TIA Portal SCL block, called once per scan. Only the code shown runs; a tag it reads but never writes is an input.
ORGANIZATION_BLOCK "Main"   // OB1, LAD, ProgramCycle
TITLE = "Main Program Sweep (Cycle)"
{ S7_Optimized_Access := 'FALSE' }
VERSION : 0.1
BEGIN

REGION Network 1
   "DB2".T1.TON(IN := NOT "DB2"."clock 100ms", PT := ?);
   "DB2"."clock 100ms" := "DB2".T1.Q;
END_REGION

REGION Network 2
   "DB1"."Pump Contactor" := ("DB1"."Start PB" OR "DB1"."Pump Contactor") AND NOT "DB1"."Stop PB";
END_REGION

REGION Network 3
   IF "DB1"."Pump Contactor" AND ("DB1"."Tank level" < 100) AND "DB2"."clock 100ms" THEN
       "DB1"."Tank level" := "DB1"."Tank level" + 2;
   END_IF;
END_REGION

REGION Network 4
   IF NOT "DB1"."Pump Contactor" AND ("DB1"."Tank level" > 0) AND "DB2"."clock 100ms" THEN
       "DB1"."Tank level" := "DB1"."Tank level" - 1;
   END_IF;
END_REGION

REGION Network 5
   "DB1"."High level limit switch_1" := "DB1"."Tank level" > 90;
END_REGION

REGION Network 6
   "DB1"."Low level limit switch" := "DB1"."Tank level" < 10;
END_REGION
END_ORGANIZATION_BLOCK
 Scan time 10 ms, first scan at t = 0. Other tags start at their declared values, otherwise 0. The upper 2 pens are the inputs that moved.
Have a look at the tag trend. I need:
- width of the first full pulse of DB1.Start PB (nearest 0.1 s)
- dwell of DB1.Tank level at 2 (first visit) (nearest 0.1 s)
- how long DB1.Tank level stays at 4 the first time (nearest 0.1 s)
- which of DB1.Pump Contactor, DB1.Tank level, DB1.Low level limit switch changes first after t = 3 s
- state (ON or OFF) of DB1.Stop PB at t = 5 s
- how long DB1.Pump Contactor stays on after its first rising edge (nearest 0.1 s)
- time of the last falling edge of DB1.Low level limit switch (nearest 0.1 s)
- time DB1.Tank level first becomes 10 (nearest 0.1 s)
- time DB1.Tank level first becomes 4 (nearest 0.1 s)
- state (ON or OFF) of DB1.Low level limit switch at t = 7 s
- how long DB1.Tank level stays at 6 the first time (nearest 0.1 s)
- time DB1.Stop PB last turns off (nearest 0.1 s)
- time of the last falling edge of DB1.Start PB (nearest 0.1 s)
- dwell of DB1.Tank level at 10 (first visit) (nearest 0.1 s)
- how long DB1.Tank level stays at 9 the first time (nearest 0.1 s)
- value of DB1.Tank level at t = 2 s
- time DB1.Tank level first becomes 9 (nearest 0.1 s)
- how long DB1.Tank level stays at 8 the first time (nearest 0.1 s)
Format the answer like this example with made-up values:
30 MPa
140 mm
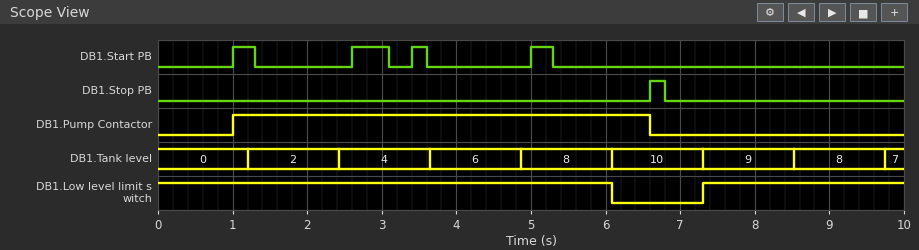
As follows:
0.3 s
1.2 s
1.2 s
DB1.Tank level
OFF
5.6 s
6.1 s
6.1 s
2.4 s
OFF
1.2 s
6.8 s
5.3 s
1.2 s
1.2 s
2
7.3 s
1.2 s
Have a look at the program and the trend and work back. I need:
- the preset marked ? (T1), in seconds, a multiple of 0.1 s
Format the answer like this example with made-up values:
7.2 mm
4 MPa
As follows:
1.2 s
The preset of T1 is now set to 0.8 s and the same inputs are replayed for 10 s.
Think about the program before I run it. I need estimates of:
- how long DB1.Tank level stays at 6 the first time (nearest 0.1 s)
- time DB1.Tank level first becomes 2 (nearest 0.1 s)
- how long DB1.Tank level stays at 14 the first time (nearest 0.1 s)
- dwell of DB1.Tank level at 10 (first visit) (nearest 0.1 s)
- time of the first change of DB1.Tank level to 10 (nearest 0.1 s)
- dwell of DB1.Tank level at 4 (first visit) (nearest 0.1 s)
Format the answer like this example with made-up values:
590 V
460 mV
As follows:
0.8 s
1.6 s
0.8 s
0.8 s
4.9 s
0.8 s
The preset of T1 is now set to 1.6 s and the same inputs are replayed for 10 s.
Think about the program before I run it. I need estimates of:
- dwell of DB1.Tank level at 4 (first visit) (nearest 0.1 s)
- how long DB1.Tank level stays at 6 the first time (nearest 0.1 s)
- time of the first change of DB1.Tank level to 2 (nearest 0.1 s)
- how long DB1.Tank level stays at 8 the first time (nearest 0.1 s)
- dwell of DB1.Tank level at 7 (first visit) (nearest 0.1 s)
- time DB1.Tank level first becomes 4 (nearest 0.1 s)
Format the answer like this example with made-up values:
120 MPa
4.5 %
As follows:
1.6 s
1.6 s
1.6 s
1.6 s
1.6 s
3.2 s
